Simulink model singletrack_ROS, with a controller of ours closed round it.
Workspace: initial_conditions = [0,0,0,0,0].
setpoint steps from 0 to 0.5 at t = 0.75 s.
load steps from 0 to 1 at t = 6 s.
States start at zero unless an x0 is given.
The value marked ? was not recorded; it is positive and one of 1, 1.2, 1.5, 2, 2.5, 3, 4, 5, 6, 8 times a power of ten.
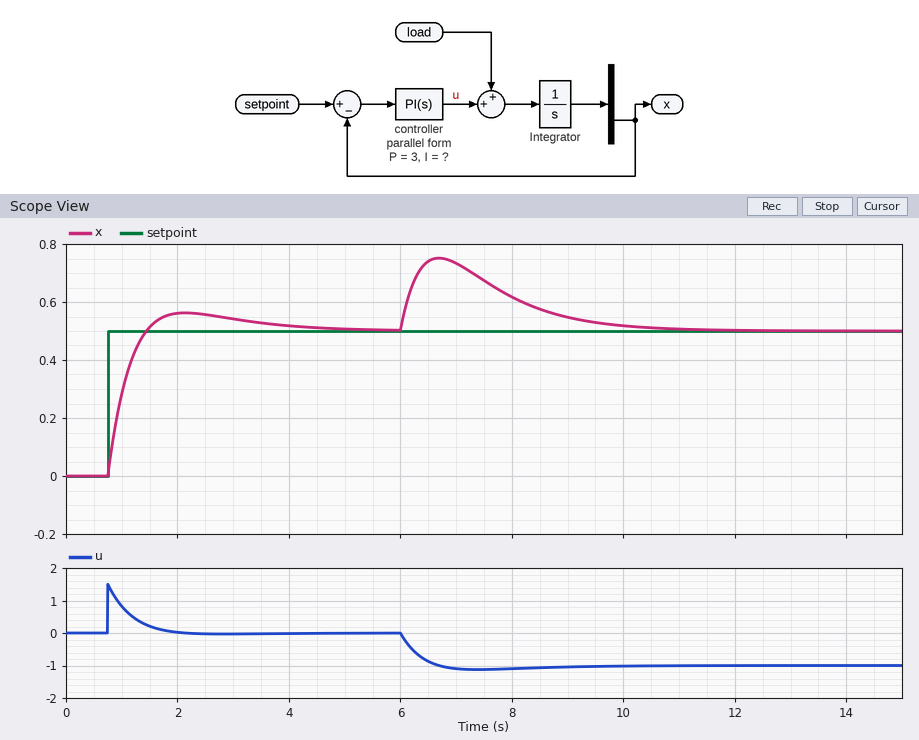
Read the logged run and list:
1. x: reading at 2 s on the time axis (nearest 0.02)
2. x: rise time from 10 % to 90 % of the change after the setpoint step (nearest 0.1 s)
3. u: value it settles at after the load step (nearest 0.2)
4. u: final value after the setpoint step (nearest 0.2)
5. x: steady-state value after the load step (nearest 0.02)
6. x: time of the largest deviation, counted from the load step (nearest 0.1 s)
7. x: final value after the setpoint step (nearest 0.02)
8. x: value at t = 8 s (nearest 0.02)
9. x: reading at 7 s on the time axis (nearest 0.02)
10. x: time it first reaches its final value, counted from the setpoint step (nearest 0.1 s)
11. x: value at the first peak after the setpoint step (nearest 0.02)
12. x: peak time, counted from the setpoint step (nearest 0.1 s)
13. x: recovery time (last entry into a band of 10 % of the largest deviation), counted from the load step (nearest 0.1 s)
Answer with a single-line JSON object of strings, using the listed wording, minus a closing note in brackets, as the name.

{"x: reading at 2 s on the time axis": "0.56", "x: rise time from 10 % to 90 % of the change after the setpoint step": "0.5 s", "u: value it settles at after the load step": "-1.0", "u: final value after the setpoint step": "0.0", "x: steady-state value after the load step": "0.50", "x: time of the largest deviation, counted from the load step": "0.7 s", "x: final value after the setpoint step": "0.50", "x: value at t = 8 s": "0.62", "x: reading at 7 s on the time axis": "0.74", "x: time it first reaches its final value, counted from the setpoint step": "0.7 s", "x: value at the first peak after the setpoint step": "0.56", "x: peak time, counted from the setpoint step": "1.4 s", "x: recovery time (last entry into a band of 10 % of the largest deviation), counted from the load step": "3.7 s"}
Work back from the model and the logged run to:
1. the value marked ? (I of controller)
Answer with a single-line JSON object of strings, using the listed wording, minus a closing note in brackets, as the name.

{"the value marked ?": "2"}
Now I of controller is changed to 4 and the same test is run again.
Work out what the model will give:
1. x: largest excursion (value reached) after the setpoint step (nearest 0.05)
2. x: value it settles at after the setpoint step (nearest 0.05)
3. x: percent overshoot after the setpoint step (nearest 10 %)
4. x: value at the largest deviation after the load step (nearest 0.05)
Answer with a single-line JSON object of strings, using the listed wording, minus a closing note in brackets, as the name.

{"x: largest excursion (value reached) after the setpoint step": "0.60", "x: value it settles at after the setpoint step": "0.50", "x: percent overshoot after the setpoint step": "20 %", "x: value at the largest deviation after the load step": "0.70"}
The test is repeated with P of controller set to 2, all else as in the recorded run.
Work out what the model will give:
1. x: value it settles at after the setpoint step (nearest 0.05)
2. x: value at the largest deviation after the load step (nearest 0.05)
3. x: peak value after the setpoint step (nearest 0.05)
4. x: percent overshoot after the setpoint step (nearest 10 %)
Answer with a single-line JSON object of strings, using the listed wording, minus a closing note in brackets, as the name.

{"x: value it settles at after the setpoint step": "0.50", "x: value at the largest deviation after the load step": "0.80", "x: peak value after the setpoint step": "0.60", "x: percent overshoot after the setpoint step": "20 %"}
